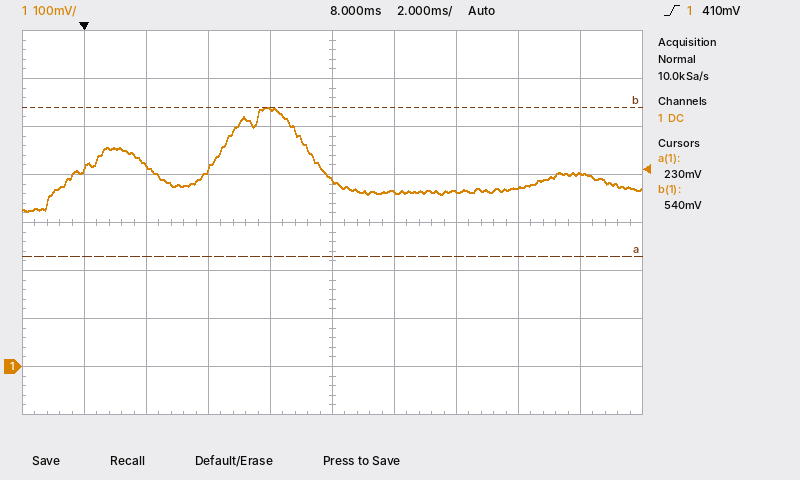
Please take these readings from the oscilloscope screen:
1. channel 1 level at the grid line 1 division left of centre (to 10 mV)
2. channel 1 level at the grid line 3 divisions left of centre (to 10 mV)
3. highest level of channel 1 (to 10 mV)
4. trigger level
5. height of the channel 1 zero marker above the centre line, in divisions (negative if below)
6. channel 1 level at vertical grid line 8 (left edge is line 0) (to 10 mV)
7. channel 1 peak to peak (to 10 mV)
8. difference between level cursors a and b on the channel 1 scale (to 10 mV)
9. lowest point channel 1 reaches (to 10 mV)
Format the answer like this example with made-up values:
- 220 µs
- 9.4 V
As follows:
- 540 mV
- 420 mV
- 540 mV
- 410 mV
- -3.0 div
- 370 mV
- 220 mV
- 310 mV
- 320 mV
